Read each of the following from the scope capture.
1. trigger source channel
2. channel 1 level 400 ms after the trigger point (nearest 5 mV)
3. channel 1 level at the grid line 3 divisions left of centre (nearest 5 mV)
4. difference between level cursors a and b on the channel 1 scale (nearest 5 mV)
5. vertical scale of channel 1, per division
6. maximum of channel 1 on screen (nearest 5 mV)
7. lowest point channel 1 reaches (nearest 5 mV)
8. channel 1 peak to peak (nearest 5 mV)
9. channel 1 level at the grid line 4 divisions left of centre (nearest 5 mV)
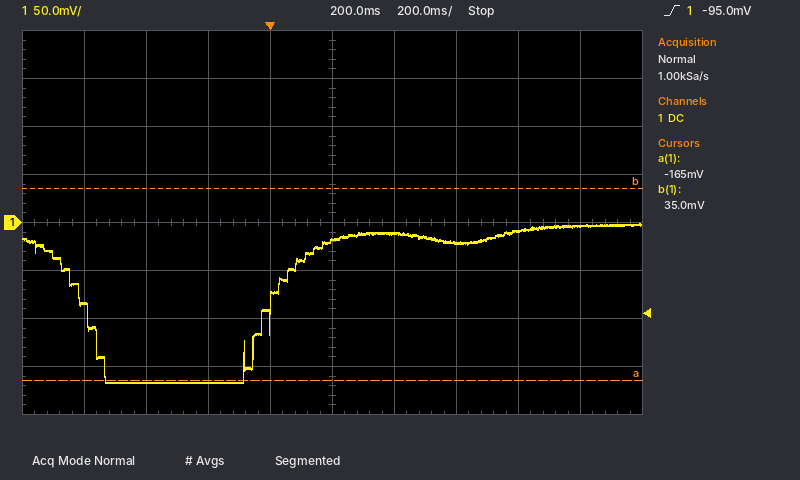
channel 1
-10 mV
-165 mV
200 mV
50 mV
0 mV
-165 mV
165 mV
-85 mV
